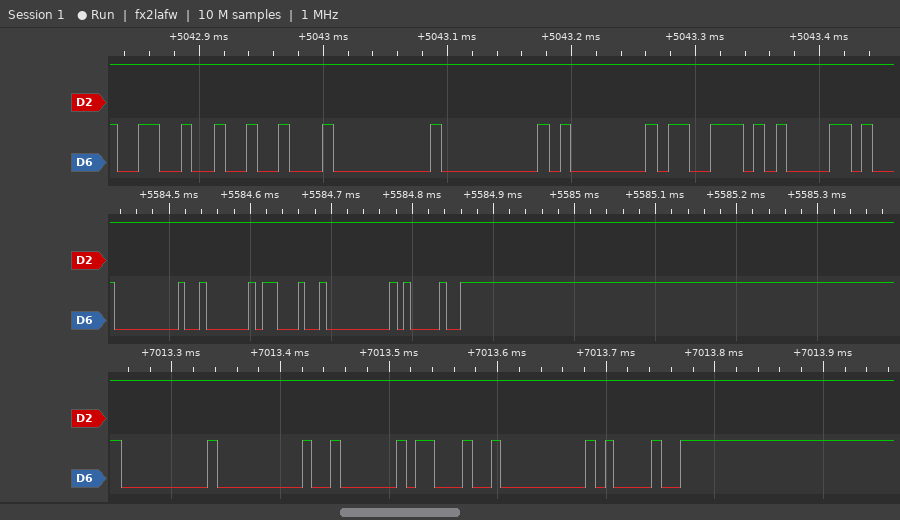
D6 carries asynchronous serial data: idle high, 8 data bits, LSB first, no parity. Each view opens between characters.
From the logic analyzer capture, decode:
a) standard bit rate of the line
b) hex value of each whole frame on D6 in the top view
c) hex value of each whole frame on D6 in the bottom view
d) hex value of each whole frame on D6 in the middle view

115200 baud
26, 12, 00, 00, 01, 73, 61
00, 00, 02, 23, 00, 21
00, 02, 23, 00, 21
